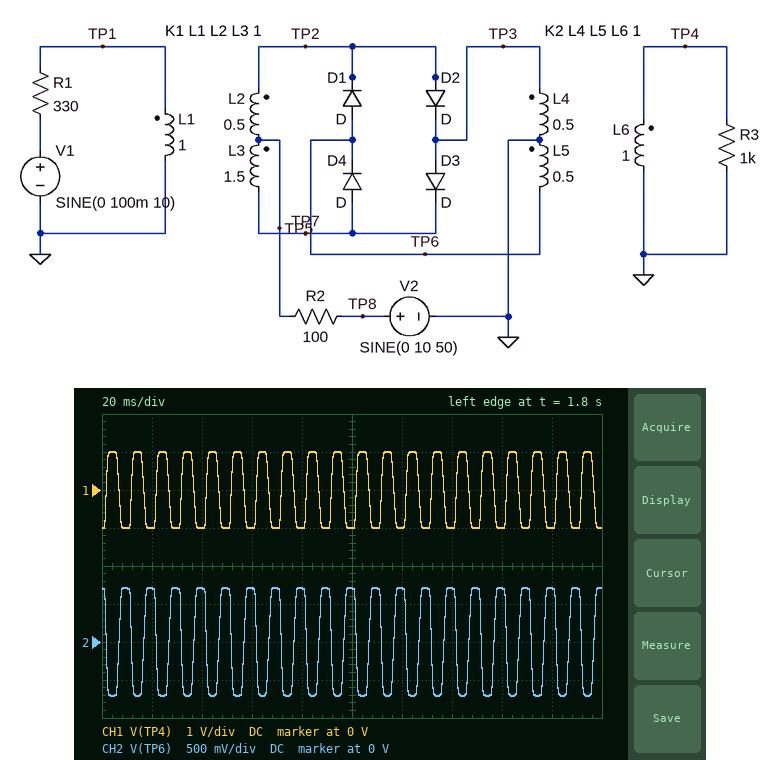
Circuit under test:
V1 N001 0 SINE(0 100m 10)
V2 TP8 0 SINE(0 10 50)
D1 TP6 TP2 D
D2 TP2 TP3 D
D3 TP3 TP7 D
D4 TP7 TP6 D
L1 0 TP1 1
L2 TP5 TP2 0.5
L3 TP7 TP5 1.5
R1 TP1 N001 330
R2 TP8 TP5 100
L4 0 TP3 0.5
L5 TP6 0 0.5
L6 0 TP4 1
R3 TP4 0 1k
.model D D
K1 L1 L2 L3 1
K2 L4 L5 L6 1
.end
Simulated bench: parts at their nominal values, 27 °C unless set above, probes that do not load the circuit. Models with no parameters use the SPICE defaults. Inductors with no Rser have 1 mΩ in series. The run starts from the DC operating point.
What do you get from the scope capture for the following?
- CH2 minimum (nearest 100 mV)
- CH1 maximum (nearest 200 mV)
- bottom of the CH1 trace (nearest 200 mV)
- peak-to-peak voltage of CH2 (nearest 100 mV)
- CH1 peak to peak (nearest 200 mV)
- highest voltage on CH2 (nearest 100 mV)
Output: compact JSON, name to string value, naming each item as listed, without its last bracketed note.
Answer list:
{"CH2 minimum": "-700 mV", "CH1 maximum": "1.0 V", "bottom of the CH1 trace": "-1.0 V", "peak-to-peak voltage of CH2": "1.4 V", "CH1 peak to peak": "2.0 V", "highest voltage on CH2": "700 mV"}
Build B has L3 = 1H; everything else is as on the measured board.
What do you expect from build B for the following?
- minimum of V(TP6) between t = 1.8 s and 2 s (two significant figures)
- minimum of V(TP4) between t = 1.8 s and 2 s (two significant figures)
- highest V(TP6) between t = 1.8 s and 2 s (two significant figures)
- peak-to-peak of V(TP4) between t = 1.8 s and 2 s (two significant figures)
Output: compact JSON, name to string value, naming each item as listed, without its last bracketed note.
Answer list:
{"minimum of V(TP6) between t = 1.8 s and 2 s": "-680 mV", "minimum of V(TP4) between t = 1.8 s and 2 s": "-980 mV", "highest V(TP6) between t = 1.8 s and 2 s": "690 mV", "peak-to-peak of V(TP4) between t = 1.8 s and 2 s": "1.9 V"}
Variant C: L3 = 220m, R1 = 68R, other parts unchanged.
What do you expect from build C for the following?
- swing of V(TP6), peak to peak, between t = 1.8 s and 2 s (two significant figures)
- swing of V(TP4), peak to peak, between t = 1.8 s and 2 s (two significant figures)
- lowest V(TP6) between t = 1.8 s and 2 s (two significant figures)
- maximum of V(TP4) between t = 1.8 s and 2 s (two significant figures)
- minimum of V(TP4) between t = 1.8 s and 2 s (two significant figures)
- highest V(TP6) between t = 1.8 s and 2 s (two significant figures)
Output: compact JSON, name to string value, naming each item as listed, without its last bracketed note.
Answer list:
{"swing of V(TP6), peak to peak, between t = 1.8 s and 2 s": "930 mV", "swing of V(TP4), peak to peak, between t = 1.8 s and 2 s": "1.3 V", "lowest V(TP6) between t = 1.8 s and 2 s": "-690 mV", "maximum of V(TP4) between t = 1.8 s and 2 s": "980 mV", "minimum of V(TP4) between t = 1.8 s and 2 s": "-340 mV", "highest V(TP6) between t = 1.8 s and 2 s": "240 mV"}
